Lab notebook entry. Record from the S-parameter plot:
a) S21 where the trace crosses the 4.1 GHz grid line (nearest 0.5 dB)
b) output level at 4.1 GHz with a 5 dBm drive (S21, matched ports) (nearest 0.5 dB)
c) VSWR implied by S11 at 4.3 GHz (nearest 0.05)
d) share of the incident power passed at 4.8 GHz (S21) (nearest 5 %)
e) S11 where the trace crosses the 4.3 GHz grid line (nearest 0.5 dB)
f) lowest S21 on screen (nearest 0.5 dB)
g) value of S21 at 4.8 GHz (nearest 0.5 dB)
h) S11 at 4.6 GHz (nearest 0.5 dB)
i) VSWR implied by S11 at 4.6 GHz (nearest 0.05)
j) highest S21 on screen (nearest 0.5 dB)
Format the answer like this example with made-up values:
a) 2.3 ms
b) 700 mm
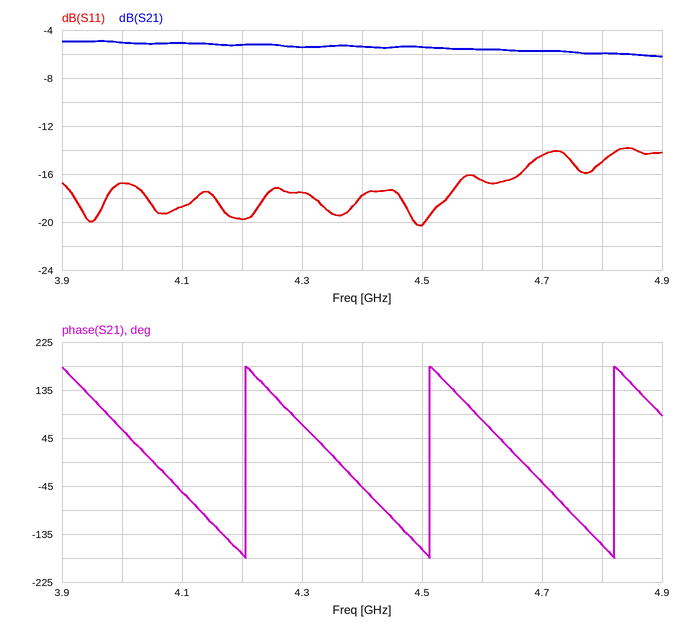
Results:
a) -5.0 dB
b) 0.0 dBm
c) 1.30
d) 25 %
e) -17.5 dB
f) -6.0 dB
g) -6.0 dB
h) -16.5 dB
i) 1.35
j) -5.0 dB
